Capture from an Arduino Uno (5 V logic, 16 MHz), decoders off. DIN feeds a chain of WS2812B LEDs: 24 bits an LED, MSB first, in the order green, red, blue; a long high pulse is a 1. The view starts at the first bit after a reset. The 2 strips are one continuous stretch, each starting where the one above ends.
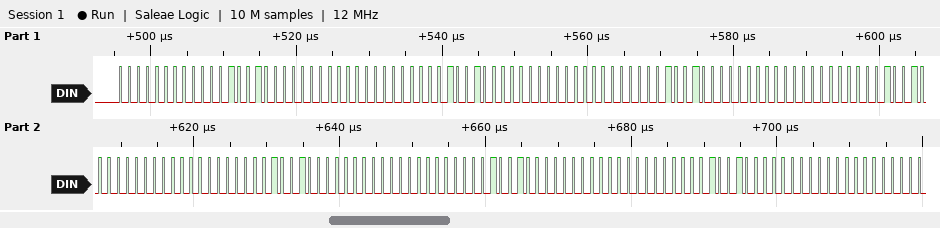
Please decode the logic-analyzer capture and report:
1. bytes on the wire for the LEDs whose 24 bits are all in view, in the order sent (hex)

00 09 00 00 09 00 00 09 00 00 09 00 00 09 00 00 09 00 00 09 00
